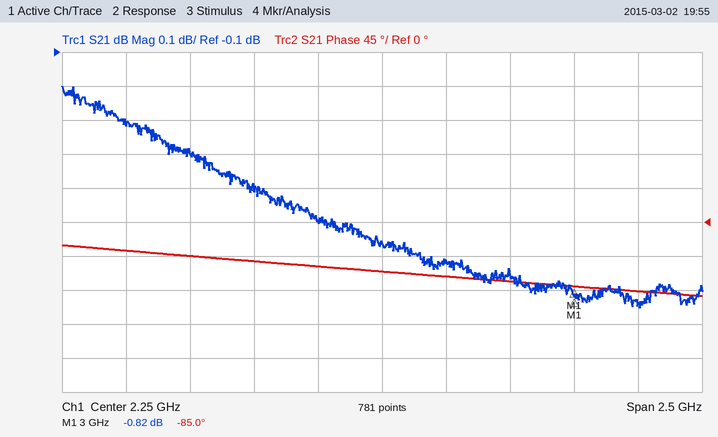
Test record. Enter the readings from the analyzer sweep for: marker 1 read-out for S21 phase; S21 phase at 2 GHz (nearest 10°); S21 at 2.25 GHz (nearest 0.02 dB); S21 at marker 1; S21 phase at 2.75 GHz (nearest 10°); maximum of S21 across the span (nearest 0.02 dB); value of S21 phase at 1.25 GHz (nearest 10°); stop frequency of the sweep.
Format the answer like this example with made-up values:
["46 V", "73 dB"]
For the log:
["-85.0°", "-60°", "-0.66 dB", "-0.82 dB", "-80°", "-0.20 dB", "-40°", "3.5 GHz"]
